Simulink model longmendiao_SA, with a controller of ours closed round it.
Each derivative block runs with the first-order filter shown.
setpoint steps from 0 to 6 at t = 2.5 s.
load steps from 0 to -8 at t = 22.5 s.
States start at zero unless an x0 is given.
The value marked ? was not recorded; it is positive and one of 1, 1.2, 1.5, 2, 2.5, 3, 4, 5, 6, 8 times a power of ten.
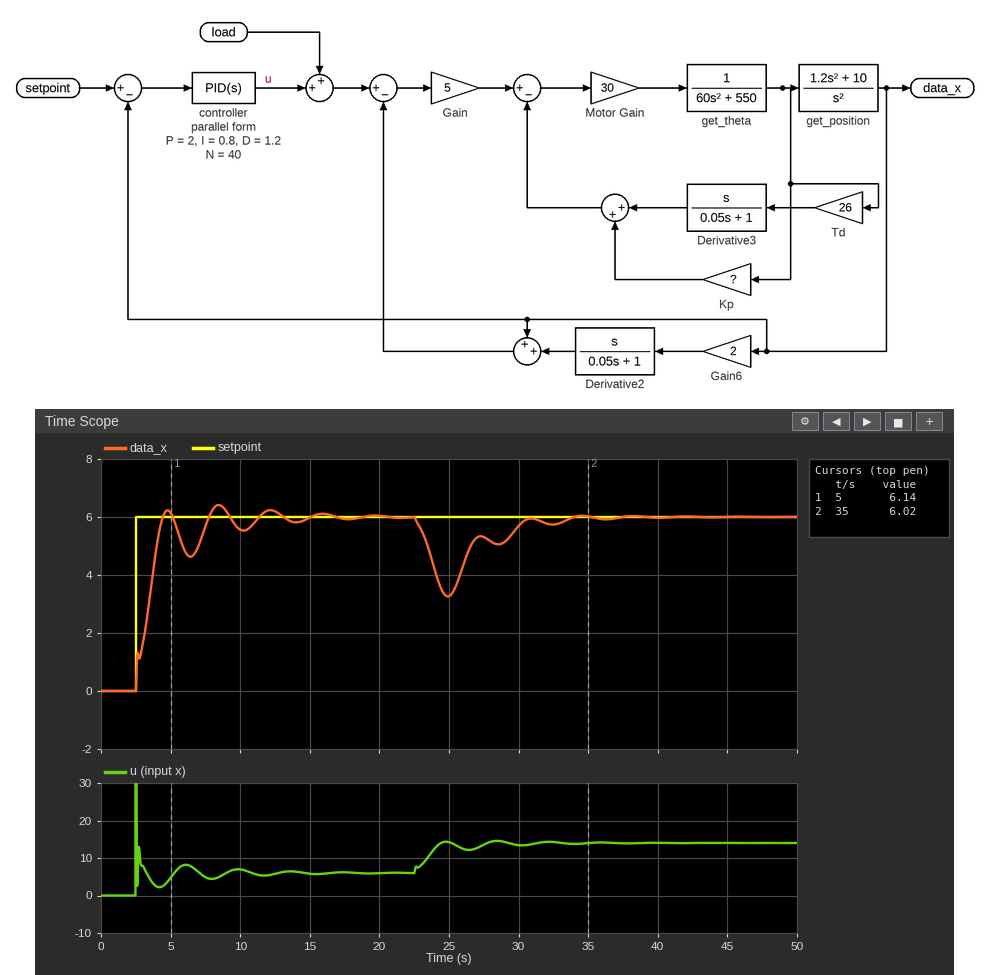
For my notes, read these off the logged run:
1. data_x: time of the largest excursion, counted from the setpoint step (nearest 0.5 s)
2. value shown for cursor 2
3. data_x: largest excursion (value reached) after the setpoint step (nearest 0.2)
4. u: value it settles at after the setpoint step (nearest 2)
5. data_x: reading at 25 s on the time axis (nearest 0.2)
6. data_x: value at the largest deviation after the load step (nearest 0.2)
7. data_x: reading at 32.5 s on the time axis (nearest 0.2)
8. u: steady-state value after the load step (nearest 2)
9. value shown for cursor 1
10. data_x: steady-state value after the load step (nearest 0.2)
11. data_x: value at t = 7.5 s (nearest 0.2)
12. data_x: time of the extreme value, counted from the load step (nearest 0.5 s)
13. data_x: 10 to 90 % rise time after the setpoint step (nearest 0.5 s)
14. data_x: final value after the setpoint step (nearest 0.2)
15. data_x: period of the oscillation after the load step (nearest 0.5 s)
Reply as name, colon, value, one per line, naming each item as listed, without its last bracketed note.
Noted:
data_x: time of the largest excursion, counted from the setpoint step: 6.0 s
value shown for cursor 2: 6.02
data_x: largest excursion (value reached) after the setpoint step: 6.4
u: value it settles at after the setpoint step: 6
data_x: reading at 25 s on the time axis: 3.2
data_x: value at the largest deviation after the load step: 3.2
data_x: reading at 32.5 s on the time axis: 5.8
u: steady-state value after the load step: 14
value shown for cursor 1: 6.14
data_x: steady-state value after the load step: 6.0
data_x: value at t = 7.5 s: 5.6
data_x: time of the extreme value, counted from the load step: 2.5 s
data_x: 10 to 90 % rise time after the setpoint step: 1.5 s
data_x: final value after the setpoint step: 6.0
data_x: period of the oscillation after the load step: 3.5 s
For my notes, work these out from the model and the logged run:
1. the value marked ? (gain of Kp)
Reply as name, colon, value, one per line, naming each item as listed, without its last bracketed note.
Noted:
the value marked ?: 40
